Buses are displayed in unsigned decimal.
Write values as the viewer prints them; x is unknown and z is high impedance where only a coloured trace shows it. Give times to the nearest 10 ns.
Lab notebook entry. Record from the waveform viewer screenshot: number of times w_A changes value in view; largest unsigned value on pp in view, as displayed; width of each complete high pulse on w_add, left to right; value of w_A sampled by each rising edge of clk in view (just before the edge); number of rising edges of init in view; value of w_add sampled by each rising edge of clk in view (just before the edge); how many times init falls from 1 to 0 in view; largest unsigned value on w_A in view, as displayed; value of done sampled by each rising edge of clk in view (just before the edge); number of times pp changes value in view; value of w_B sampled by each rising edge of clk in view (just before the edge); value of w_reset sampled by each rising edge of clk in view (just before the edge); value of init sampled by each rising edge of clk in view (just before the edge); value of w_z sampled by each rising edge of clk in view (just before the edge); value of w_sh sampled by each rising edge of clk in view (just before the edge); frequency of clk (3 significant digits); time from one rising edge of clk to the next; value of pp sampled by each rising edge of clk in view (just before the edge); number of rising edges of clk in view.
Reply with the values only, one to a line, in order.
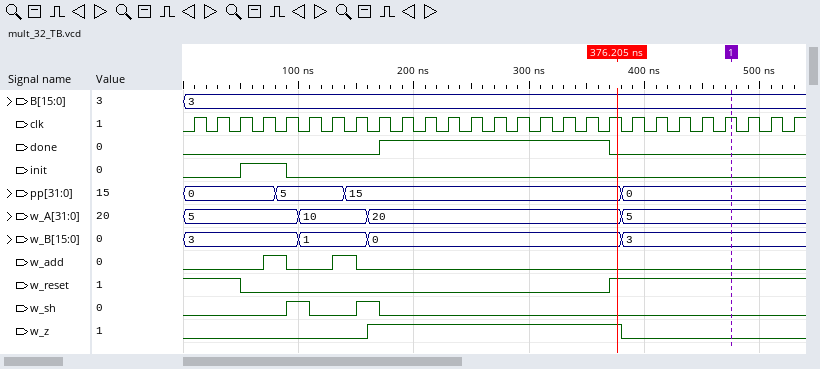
3
15
20 ns, 20 ns
5, 5, 5, 5, 5, 10, 10, 10, 20, 20, 20, 20, 20, 20, 20, 20, 20, 20, 20, 5, 5, 5, 5, 5, 5, 5, 5
1
0 0 0 0 1 0 0 1 0 0 0 0 0 0 0 0 0 0 0 0 0 0 0 0 0 0 0
1
20
0 0 0 0 0 0 0 0 0 1 1 1 1 1 1 1 1 1 1 0 0 0 0 0 0 0 0
3
3, 3, 3, 3, 3, 1, 1, 1, 0, 0, 0, 0, 0, 0, 0, 0, 0, 0, 0, 3, 3, 3, 3, 3, 3, 3, 3
1 1 1 0 0 0 0 0 0 0 0 0 0 0 0 0 0 0 0 1 1 1 1 1 1 1 1
0 0 0 1 1 0 0 0 0 0 0 0 0 0 0 0 0 0 0 0 0 0 0 0 0 0 0
0 0 0 0 0 0 0 0 1 1 1 1 1 1 1 1 1 1 1 0 0 0 0 0 0 0 0
0 0 0 0 0 1 0 0 1 0 0 0 0 0 0 0 0 0 0 0 0 0 0 0 0 0 0
50.0 MHz
20 ns
0, 0, 0, 0, 5, 5, 5, 15, 15, 15, 15, 15, 15, 15, 15, 15, 15, 15, 15, 0, 0, 0, 0, 0, 0, 0, 0
27
